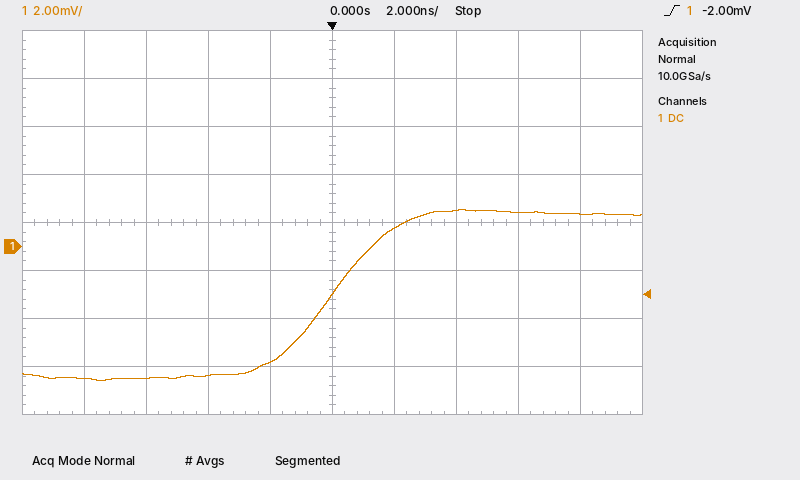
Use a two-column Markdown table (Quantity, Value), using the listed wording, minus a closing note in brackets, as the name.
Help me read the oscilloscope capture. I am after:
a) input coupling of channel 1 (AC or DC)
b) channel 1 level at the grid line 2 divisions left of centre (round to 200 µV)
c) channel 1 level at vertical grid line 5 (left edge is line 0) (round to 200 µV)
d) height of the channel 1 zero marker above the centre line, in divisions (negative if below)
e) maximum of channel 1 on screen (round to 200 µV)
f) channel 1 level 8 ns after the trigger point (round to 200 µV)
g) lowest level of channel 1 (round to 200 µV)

| Quantity | Value |
|---|---|
| input coupling of channel 1 | DC |
| channel 1 level at the grid line 2 divisions left of centre | -5.4 mV |
| channel 1 level at vertical grid line 5 (left edge is line 0) | -2.0 mV |
| height of the channel 1 zero marker above the centre line, in divisions | -0.5 div |
| maximum of channel 1 on screen | 1.6 mV |
| channel 1 level 8 ns after the trigger point | 1.4 mV |
| lowest level of channel 1 | -5.6 mV |
